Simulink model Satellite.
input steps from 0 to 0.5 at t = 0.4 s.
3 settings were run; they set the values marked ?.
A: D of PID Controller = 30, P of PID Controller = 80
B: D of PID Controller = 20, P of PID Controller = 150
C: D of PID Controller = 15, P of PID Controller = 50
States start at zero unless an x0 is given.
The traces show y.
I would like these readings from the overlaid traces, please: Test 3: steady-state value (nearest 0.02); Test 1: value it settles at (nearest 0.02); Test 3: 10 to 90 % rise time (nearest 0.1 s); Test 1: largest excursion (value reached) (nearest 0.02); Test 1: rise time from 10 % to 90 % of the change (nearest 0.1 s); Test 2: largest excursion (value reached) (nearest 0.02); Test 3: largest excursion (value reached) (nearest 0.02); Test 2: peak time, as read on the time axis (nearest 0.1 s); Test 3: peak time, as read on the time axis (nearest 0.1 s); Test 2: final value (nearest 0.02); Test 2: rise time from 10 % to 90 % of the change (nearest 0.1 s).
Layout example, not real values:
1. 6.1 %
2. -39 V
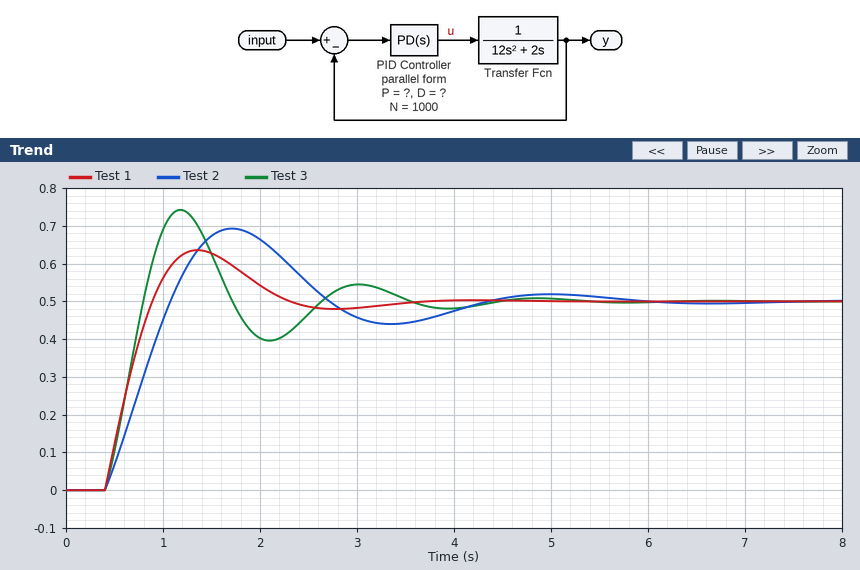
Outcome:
1. 0.50
2. 0.50
3. 0.3 s
4. 0.64
5. 0.4 s
6. 0.70
7. 0.74
8. 1.7 s
9. 1.2 s
10. 0.50
11. 0.5 s
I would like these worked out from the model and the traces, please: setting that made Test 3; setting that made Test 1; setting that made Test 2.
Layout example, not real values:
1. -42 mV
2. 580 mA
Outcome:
1. B
2. A
3. C
